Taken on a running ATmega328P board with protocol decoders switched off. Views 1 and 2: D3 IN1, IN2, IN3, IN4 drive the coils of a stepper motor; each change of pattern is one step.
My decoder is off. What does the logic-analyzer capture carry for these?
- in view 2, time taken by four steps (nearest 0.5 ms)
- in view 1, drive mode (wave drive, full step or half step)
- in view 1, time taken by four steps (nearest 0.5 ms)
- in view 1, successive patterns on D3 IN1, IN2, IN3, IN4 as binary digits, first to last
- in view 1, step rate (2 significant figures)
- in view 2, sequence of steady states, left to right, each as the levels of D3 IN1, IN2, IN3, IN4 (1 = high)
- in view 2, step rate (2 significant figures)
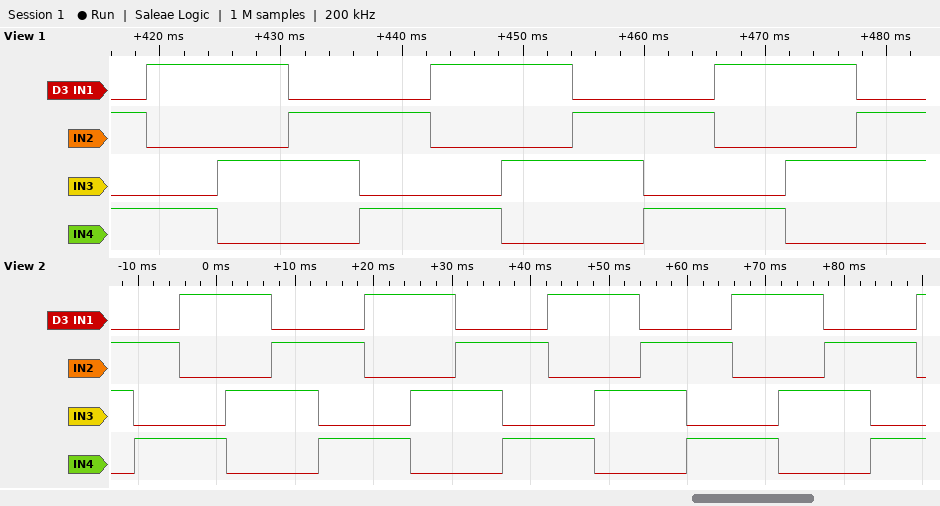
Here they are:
23.5 ms
full step
23.5 ms
0101 1001 1010 0110 0101 1001 1010 0110 0101 1001 1010 0110
170 steps/s
0110 0101 1001 1010 0110 0101 1001 1010 0110 0101 1001 1010 0110 0101 1001 1010 0110 0101 1001
170 steps/s
